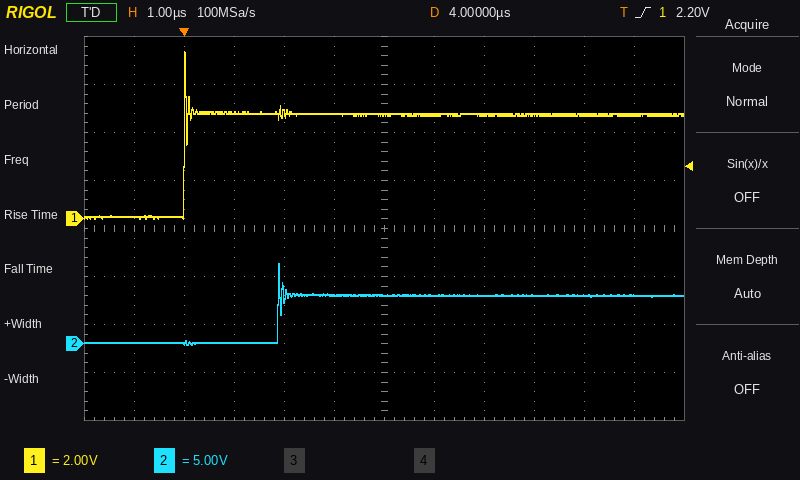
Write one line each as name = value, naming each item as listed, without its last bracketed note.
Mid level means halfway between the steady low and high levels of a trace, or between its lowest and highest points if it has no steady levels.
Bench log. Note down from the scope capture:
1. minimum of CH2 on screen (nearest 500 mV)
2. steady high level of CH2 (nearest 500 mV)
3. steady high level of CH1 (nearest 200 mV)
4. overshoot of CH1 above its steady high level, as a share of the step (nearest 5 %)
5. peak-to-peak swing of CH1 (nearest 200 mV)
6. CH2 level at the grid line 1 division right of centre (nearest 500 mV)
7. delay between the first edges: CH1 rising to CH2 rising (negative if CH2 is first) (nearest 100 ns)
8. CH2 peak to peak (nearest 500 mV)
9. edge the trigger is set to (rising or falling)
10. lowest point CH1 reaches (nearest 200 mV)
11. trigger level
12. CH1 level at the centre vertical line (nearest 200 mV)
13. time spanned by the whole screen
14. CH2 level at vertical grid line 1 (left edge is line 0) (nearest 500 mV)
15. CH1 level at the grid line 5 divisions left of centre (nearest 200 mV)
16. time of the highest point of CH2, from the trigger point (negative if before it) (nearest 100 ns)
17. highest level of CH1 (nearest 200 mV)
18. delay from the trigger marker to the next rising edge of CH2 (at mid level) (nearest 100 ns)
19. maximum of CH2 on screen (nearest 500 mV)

minimum of CH2 on screen = 0.0 V
steady high level of CH2 = 5.0 V
steady high level of CH1 = 4.4 V
overshoot of CH1 above its steady high level, as a share of the step = 60 %
peak-to-peak swing of CH1 = 7.0 V
CH2 level at the grid line 1 division right of centre = 5.0 V
delay between the first edges: CH1 rising to CH2 rising (negative if CH2 is first) = +1.9 µs
CH2 peak to peak = 8.5 V
edge the trigger is set to = rising
lowest point CH1 reaches = 0.0 V
trigger level = 2.20 V
CH1 level at the centre vertical line = 4.4 V
time spanned by the whole screen = 12 µs
CH2 level at vertical grid line 1 (left edge is line 0) = 0.0 V
CH1 level at the grid line 5 divisions left of centre = 0.0 V
time of the highest point of CH2, from the trigger point (negative if before it) = +1.9 µs
highest level of CH1 = 7.0 V
delay from the trigger marker to the next rising edge of CH2 (at mid level) = 1.9 µs
maximum of CH2 on screen = 8.5 V
